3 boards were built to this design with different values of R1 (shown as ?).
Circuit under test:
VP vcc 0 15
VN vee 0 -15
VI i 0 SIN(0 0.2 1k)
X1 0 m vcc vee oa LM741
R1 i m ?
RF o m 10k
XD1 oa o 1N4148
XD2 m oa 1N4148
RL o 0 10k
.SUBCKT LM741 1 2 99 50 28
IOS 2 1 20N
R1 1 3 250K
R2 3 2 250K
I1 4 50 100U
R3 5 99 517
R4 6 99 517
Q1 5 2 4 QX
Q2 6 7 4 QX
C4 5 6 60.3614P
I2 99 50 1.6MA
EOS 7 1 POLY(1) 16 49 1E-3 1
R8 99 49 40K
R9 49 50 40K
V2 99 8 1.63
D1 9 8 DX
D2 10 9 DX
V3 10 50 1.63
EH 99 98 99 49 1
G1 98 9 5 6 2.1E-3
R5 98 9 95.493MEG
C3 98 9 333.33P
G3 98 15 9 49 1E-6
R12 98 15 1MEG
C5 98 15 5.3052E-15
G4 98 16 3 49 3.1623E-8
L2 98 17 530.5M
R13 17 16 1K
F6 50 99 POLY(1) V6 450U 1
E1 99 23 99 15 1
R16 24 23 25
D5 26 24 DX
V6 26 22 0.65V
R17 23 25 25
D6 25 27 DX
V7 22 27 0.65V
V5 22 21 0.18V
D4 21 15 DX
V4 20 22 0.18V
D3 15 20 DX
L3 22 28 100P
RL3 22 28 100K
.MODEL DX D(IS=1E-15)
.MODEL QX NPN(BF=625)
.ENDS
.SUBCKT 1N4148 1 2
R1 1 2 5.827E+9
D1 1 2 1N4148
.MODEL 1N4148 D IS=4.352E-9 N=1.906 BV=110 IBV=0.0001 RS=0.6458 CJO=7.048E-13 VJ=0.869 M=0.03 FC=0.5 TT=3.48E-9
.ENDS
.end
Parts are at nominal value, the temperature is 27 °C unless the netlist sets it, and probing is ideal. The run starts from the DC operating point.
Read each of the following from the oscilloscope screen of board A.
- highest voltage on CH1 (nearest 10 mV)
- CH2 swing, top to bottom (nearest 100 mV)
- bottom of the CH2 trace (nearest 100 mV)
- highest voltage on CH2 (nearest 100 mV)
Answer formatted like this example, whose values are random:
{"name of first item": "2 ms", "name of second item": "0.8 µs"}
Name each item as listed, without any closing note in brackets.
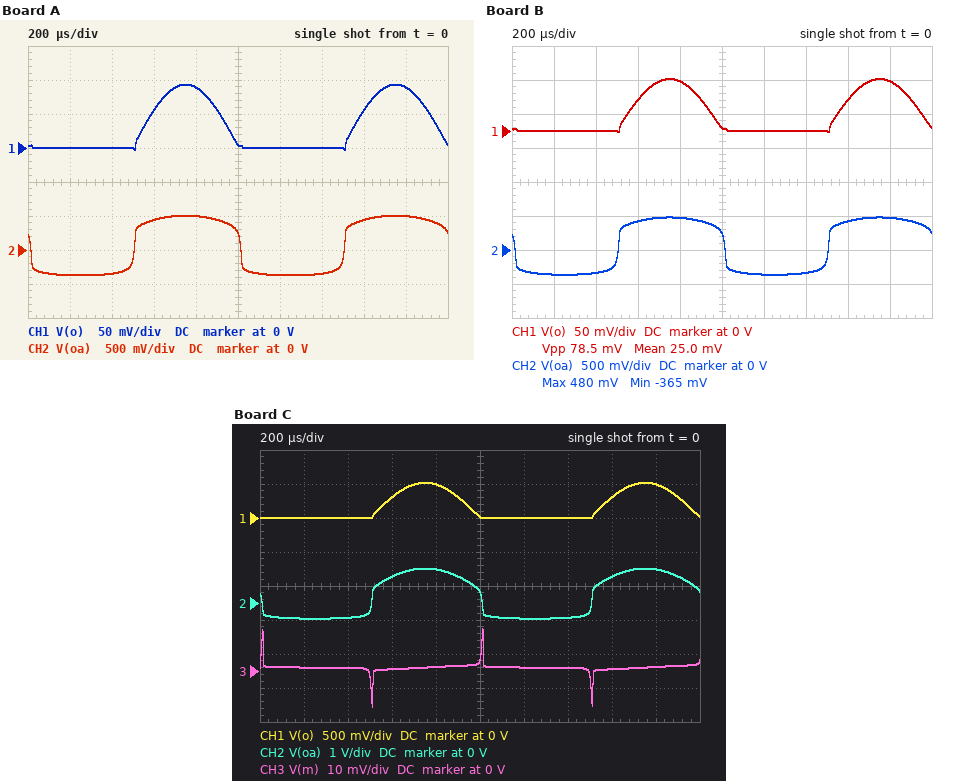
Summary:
{"highest voltage on CH1": "90 mV", "CH2 swing, top to bottom": "900 mV", "bottom of the CH2 trace": "-400 mV", "highest voltage on CH2": "500 mV"}
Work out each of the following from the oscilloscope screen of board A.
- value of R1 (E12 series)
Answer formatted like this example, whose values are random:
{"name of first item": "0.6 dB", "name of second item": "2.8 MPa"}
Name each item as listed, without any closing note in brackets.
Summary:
{"value of R1": "22 kΩ"}
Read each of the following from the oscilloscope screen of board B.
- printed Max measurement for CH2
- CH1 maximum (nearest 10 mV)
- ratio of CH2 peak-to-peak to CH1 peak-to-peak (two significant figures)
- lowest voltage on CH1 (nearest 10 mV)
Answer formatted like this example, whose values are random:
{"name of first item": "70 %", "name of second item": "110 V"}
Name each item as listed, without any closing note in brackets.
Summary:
{"printed Max measurement for CH2": "480 mV", "CH1 maximum": "80 mV", "ratio of CH2 peak-to-peak to CH1 peak-to-peak": "11", "lowest voltage on CH1": "0 V"}
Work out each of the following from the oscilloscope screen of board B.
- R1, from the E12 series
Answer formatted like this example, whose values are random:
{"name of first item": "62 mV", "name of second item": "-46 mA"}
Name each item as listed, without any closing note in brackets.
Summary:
{"R1, from the E12 series": "27 kΩ"}
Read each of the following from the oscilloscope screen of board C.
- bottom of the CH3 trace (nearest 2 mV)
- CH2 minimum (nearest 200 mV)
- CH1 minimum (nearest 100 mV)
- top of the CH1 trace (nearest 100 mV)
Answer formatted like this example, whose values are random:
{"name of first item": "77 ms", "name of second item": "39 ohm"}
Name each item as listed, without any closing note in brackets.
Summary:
{"bottom of the CH3 trace": "-10 mV", "CH2 minimum": "-400 mV", "CH1 minimum": "0 V", "top of the CH1 trace": "500 mV"}
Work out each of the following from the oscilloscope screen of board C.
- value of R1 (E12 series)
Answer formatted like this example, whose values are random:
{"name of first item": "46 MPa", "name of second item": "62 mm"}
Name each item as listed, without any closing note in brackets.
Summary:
{"value of R1": "3.9 kΩ"}
